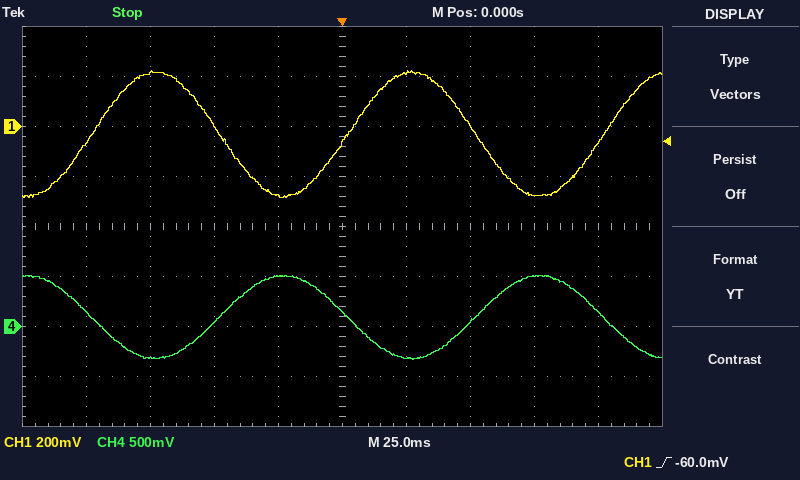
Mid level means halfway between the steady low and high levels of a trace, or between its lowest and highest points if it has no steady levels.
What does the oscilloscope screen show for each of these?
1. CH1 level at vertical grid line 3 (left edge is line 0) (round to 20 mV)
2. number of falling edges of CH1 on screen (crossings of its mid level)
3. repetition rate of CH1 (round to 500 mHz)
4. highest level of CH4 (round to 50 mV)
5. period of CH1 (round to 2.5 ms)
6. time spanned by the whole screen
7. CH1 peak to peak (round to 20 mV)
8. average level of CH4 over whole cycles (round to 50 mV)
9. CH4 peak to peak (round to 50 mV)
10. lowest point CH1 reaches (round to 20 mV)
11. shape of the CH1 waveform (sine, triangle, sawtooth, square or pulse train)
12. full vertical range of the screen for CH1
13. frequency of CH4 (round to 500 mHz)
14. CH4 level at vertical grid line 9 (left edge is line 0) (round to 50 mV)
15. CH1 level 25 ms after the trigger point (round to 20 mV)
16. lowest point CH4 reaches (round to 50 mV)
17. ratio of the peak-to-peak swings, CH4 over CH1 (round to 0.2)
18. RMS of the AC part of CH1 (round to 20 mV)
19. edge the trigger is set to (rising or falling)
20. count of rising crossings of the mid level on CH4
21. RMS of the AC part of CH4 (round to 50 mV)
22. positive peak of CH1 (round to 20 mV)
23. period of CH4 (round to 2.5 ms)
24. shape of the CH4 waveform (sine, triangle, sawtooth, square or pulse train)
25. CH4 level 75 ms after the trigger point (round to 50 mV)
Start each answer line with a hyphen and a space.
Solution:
- 0 mV
- 2
- 10.0 Hz
- 500 mV
- 100.0 ms
- 250 ms
- 500 mV
- 100 mV
- 850 mV
- -280 mV
- sine
- 1.6 V
- 10.0 Hz
- 150 mV
- 220 mV
- -350 mV
- 1.6
- 180 mV
- rising
- 2
- 300 mV
- 220 mV
- 100.0 ms
- sine
- 500 mV
